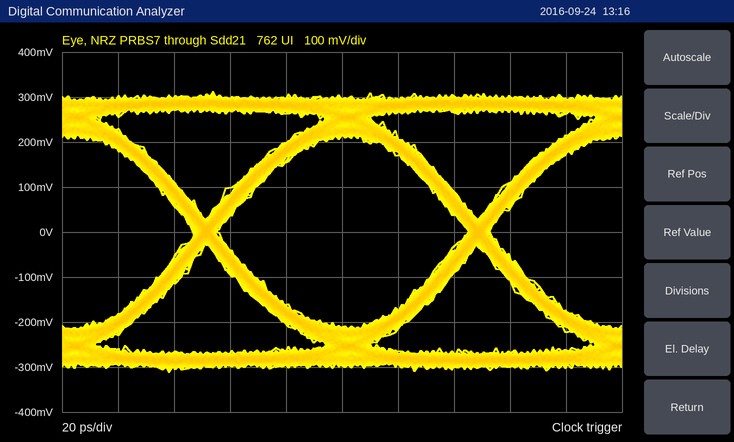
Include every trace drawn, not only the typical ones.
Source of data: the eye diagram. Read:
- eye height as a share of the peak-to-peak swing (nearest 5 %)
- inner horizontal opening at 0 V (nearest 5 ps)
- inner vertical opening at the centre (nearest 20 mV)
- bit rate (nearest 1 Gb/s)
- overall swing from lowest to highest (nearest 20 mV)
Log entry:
70 %
90 ps
420 mV
10 Gb/s
620 mV
